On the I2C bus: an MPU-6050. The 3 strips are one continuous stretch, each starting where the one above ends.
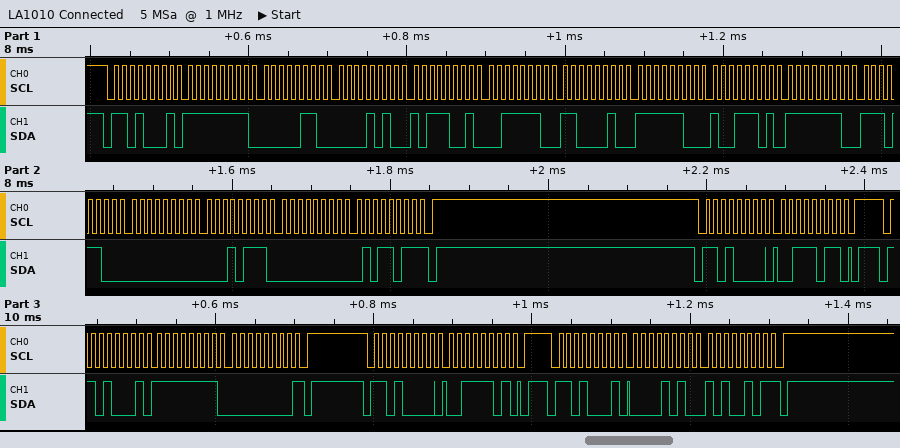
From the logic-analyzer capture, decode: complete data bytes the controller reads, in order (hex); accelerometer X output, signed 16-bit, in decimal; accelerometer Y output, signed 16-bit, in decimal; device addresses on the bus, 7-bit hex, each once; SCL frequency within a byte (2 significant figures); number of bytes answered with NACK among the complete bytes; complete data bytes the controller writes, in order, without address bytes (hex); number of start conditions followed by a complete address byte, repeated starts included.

FF 06 0A B9 3E C2 FC 9D FE EC 00 17 00 5B FF 00 0A A5
-256
2725
0x68
100 kHz
3
3B 3D
5
